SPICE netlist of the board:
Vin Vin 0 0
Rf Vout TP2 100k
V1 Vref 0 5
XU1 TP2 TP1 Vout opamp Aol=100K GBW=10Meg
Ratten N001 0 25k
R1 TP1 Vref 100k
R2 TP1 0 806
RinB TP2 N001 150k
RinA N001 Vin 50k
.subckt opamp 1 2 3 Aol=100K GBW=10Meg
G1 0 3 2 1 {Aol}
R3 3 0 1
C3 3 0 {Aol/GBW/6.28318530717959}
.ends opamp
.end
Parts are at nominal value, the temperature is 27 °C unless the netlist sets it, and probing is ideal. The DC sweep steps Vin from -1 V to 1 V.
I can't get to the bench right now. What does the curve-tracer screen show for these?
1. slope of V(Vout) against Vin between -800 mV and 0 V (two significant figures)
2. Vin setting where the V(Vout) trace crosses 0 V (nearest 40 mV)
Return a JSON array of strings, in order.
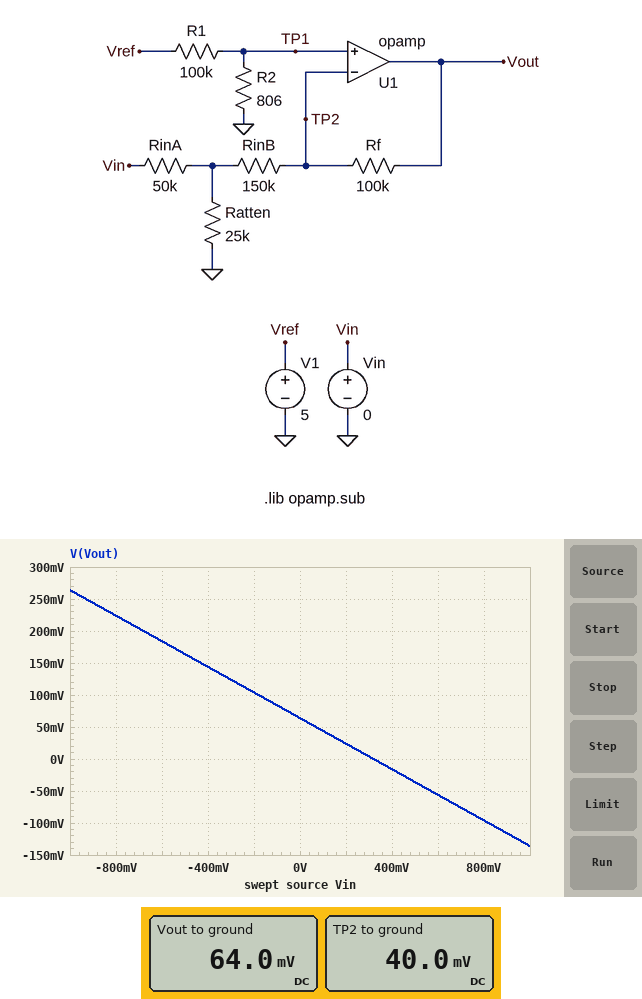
["-0.20 V/V", "320 mV"]
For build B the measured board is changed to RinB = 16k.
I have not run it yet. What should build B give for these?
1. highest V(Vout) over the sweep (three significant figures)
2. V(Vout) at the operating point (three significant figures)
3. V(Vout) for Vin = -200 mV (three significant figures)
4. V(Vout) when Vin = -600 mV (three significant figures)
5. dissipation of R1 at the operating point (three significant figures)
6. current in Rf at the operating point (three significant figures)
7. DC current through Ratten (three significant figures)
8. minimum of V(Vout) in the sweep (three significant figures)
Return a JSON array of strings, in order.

["1.18 V", "162 mV", "366 mV", "775 mV", "246 µW", "1.22 µA", "816 nA", "-858 mV"]
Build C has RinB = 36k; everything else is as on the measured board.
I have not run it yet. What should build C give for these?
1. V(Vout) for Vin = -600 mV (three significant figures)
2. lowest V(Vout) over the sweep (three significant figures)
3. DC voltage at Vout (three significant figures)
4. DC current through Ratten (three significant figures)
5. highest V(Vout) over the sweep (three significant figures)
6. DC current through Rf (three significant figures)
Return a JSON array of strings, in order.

["496 mV", "-517 mV", "116 mV", "506 nA", "749 mV", "759 nA"]
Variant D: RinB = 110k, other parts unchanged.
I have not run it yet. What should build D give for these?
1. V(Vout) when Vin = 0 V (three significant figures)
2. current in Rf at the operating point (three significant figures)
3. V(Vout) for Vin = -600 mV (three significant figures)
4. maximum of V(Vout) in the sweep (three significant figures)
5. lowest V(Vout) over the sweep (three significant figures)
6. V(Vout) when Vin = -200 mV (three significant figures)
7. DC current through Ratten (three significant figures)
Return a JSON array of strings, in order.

["71.5 mV", "316 nA", "229 mV", "335 mV", "-192 mV", "124 mV", "210 nA"]
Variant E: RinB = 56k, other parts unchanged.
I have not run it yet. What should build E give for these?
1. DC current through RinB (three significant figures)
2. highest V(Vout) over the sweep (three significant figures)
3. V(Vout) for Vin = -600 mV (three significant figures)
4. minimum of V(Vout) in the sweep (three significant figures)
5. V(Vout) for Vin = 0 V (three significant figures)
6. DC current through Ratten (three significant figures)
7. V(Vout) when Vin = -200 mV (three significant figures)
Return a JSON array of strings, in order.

["550 nA", "554 mV", "370 mV", "-364 mV", "95.0 mV", "367 nA", "187 mV"]
